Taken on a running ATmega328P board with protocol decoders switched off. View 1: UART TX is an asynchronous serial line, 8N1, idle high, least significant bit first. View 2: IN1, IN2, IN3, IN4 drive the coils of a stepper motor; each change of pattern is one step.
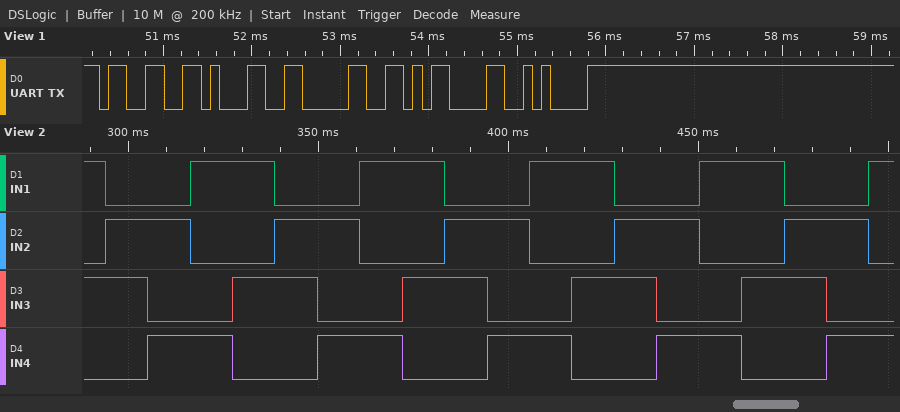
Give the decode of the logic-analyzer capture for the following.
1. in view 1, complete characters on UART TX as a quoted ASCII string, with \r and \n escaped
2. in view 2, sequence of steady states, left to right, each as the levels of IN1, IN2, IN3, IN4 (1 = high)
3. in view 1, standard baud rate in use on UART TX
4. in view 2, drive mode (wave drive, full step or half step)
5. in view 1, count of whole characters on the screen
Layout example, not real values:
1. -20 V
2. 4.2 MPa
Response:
1. "310\r\n"
2. 1010 0110 0101 1001 1010 0110 0101 1001 1010 0110 0101 1001 1010 0110 0101 1001 1010 0110 0101 1001
3. 9600 baud
4. full step
5. 5
